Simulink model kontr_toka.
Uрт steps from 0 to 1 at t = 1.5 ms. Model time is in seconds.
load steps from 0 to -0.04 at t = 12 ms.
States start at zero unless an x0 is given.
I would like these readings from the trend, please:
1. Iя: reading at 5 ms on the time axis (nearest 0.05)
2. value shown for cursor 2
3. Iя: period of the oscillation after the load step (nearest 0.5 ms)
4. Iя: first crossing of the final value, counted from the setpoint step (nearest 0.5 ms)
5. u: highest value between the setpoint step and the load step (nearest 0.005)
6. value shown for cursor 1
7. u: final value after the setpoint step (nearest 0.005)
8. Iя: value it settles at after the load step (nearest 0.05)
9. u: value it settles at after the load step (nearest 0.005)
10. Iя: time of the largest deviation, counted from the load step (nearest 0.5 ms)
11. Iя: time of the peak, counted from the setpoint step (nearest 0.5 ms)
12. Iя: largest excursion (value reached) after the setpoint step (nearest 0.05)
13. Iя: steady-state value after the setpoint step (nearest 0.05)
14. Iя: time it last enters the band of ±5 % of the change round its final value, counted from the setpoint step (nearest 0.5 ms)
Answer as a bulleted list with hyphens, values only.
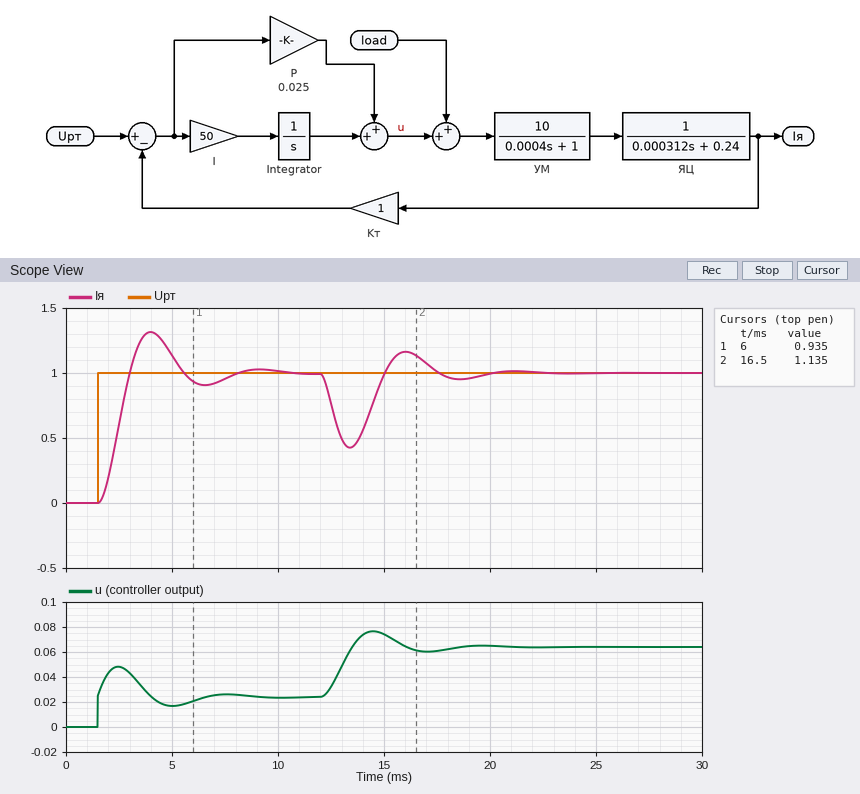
- 1.15
- 1.135
- 5.0 ms
- 1.5 ms
- 0.050
- 0.935
- 0.025
- 1.00
- 0.065
- 1.5 ms
- 2.5 ms
- 1.30
- 1.00
- 6.0 ms
